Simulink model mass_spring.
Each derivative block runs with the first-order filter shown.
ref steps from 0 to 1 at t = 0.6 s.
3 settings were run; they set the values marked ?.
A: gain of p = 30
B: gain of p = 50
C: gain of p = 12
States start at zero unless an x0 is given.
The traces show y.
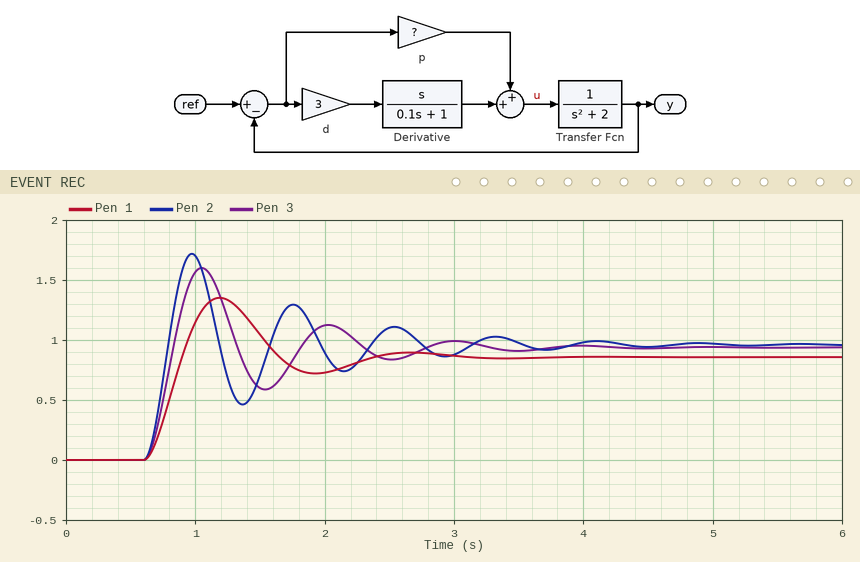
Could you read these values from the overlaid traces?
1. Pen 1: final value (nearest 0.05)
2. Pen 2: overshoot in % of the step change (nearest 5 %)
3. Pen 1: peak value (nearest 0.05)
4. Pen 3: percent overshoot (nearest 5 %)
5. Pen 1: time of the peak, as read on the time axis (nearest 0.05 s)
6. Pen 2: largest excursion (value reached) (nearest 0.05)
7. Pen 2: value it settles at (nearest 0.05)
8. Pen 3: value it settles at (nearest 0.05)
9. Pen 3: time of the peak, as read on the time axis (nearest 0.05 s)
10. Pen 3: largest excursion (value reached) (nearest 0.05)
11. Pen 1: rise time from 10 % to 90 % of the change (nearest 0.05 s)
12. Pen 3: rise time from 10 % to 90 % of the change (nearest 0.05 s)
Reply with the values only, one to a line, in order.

0.85
80 %
1.35
70 %
1.20 s
1.70
0.95
0.95
1.05 s
1.60
0.20 s
0.15 s
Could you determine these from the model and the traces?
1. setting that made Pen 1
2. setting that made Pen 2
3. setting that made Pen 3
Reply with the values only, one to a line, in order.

C
B
A
